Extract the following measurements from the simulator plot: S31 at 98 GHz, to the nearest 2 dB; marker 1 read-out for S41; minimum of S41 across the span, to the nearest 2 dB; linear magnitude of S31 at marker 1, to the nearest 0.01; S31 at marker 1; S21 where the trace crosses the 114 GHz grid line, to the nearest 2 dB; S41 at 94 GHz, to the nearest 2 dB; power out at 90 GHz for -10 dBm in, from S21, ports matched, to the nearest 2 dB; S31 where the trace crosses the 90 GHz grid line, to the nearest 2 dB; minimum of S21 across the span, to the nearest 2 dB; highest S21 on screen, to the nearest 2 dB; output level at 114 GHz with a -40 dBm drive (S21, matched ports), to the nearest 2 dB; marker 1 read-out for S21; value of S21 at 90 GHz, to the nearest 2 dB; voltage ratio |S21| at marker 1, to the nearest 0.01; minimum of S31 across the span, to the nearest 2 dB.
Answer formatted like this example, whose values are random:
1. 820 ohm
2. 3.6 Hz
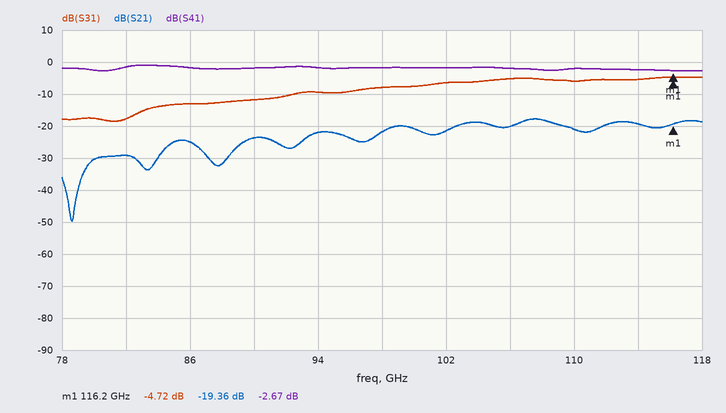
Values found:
1. -8 dB
2. -2.67 dB
3. -2 dB
4. 0.58
5. -4.72 dB
6. -20 dB
7. -2 dB
8. -34 dBm
9. -12 dB
10. -50 dB
11. -18 dB
12. -60 dBm
13. -19.36 dB
14. -24 dB
15. 0.11
16. -18 dB
